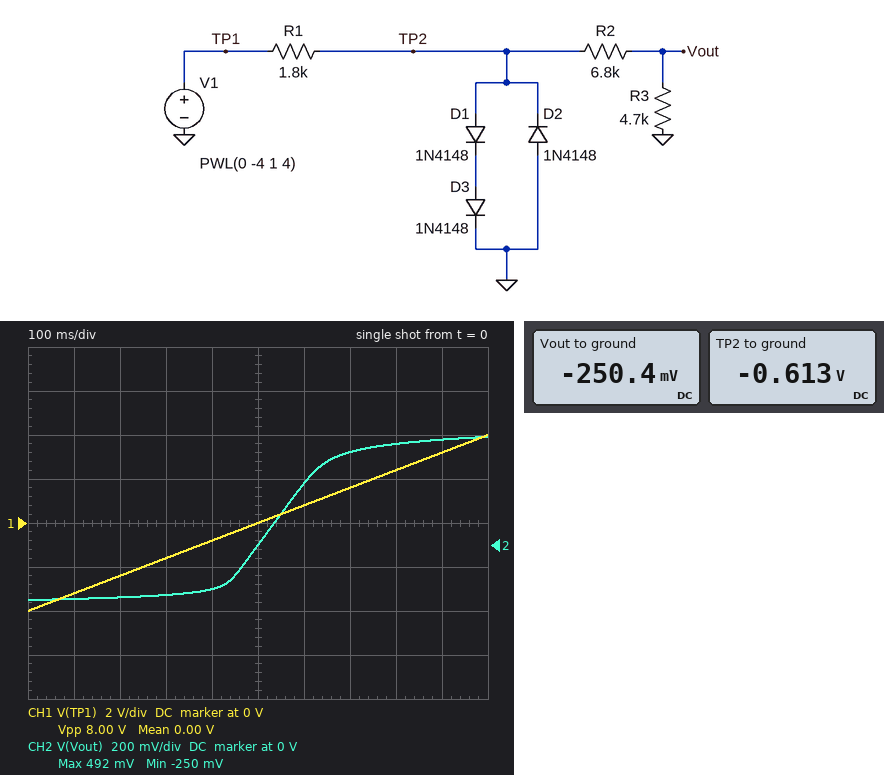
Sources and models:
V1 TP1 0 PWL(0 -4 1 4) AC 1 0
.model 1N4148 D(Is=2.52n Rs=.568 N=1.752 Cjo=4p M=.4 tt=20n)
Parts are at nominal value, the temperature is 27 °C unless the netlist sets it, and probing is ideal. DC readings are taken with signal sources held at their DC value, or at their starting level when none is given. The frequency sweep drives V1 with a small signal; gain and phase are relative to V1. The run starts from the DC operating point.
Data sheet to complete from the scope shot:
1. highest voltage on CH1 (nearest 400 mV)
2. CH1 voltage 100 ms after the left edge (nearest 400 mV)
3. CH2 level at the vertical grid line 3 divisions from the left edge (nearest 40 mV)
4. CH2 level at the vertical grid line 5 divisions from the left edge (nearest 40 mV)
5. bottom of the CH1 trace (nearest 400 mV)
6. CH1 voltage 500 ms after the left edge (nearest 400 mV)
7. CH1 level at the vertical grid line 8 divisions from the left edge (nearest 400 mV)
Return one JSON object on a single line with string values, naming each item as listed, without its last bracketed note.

{"highest voltage on CH1": "4.0 V", "CH1 voltage 100 ms after the left edge": "-3.2 V", "CH2 level at the vertical grid line 3 divisions from the left edge": "-240 mV", "CH2 level at the vertical grid line 5 divisions from the left edge": "0 V", "bottom of the CH1 trace": "-4.0 V", "CH1 voltage 500 ms after the left edge": "0 V", "CH1 level at the vertical grid line 8 divisions from the left edge": "2.4 V"}
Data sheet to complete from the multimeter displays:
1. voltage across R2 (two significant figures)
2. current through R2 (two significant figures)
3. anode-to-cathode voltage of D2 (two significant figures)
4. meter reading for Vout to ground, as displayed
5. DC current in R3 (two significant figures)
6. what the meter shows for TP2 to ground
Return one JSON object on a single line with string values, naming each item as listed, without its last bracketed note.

{"voltage across R2": "360 mV", "current through R2": "53 µA", "anode-to-cathode voltage of D2": "610 mV", "meter reading for Vout to ground, as displayed": "-250.4 mV", "DC current in R3": "53 µA", "what the meter shows for TP2 to ground": "-0.613 V"}
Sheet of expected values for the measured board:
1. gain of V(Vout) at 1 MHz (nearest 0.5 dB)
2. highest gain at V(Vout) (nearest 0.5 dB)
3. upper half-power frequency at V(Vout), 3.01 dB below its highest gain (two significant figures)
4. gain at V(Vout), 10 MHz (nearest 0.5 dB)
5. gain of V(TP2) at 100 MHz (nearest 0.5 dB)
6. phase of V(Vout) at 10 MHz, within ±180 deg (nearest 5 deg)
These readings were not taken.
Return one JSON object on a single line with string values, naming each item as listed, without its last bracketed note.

{"gain of V(Vout) at 1 MHz": "-45.0 dB", "highest gain at V(Vout)": "-45.0 dB", "upper half-power frequency at V(Vout), 3.01 dB below its highest gain": "8.0 MHz", "gain at V(Vout), 10 MHz": "-49.0 dB", "gain of V(TP2) at 100 MHz": "-59.0 dB", "phase of V(Vout) at 10 MHz, within ±180 deg": "-50 deg"}
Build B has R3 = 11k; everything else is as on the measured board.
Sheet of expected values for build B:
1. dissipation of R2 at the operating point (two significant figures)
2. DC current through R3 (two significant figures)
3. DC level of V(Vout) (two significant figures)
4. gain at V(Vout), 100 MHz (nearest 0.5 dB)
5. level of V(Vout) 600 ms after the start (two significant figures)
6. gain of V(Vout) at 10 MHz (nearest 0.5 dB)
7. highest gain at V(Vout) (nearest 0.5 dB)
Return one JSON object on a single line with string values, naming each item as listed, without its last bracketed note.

{"dissipation of R2 at the operating point": "8.1 µW", "DC current through R3": "34 µA", "DC level of V(Vout)": "-380 mV", "gain at V(Vout), 100 MHz": "-63.0 dB", "level of V(Vout) 600 ms after the start": "440 mV", "gain of V(Vout) at 10 MHz": "-45.5 dB", "highest gain at V(Vout)": "-41.5 dB"}
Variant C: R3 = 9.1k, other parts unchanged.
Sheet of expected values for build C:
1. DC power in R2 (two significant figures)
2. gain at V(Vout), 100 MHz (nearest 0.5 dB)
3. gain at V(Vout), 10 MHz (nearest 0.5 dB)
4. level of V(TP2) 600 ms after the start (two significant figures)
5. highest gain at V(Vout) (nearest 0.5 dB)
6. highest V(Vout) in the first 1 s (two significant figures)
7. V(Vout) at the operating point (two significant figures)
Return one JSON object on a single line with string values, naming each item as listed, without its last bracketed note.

{"DC power in R2": "10 µW", "gain at V(Vout), 100 MHz": "-63.5 dB", "gain at V(Vout), 10 MHz": "-46.0 dB", "level of V(TP2) 600 ms after the start": "710 mV", "highest gain at V(Vout)": "-42.0 dB", "highest V(Vout) in the first 1 s": "690 mV", "V(Vout) at the operating point": "-350 mV"}
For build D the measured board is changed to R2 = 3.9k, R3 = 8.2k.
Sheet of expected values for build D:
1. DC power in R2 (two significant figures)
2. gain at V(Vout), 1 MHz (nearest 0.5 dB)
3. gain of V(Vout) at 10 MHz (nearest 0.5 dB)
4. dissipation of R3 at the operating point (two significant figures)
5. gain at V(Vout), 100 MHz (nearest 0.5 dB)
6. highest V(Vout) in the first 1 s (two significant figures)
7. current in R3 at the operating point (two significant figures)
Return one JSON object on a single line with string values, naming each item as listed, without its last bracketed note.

{"DC power in R2": "10 µW", "gain at V(Vout), 1 MHz": "-40.5 dB", "gain of V(Vout) at 10 MHz": "-44.5 dB", "dissipation of R3 at the operating point": "21 µW", "gain at V(Vout), 100 MHz": "-62.0 dB", "highest V(Vout) in the first 1 s": "820 mV", "current in R3 at the operating point": "51 µA"}
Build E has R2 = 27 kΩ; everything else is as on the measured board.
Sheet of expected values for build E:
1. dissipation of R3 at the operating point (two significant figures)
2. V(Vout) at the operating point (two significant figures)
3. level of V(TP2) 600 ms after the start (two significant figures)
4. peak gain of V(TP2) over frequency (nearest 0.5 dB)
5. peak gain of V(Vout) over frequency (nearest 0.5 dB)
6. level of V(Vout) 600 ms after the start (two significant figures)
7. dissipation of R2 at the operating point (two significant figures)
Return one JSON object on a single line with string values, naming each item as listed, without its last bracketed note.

{"dissipation of R3 at the operating point": "1.8 µW", "V(Vout) at the operating point": "-91 mV", "level of V(TP2) 600 ms after the start": "740 mV", "peak gain of V(TP2) over frequency": "-37.5 dB", "peak gain of V(Vout) over frequency": "-54.0 dB", "level of V(Vout) 600 ms after the start": "110 mV", "dissipation of R2 at the operating point": "10 µW"}
